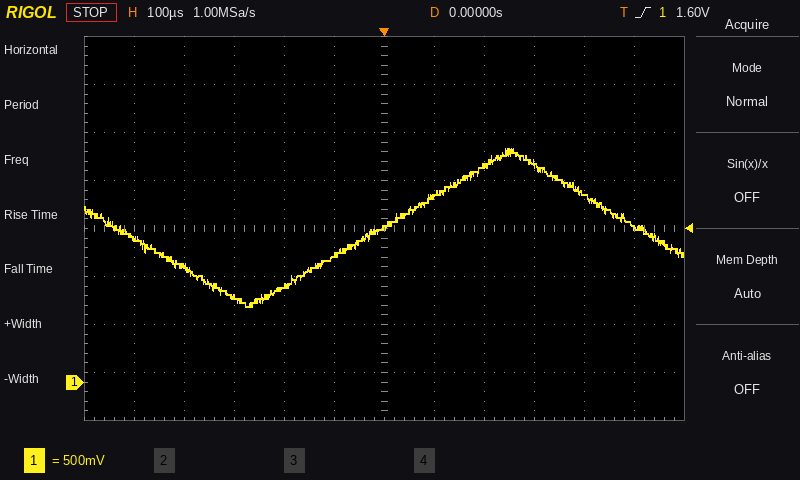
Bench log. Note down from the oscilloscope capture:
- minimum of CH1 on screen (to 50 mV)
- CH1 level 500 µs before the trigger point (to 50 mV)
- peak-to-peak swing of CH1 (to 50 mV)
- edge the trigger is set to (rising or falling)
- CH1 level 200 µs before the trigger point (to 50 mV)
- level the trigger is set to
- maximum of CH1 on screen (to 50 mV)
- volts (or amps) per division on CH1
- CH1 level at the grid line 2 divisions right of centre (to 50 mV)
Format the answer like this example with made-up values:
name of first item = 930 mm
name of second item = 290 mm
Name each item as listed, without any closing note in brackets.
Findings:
minimum of CH1 on screen = 800 mV
CH1 level 500 µs before the trigger point = 1.50 V
peak-to-peak swing of CH1 = 1.65 V
edge the trigger is set to = rising
CH1 level 200 µs before the trigger point = 1.00 V
level the trigger is set to = 1.60 V
maximum of CH1 on screen = 2.45 V
volts (or amps) per division on CH1 = 500 mV
CH1 level at the grid line 2 divisions right of centre = 2.25 V
